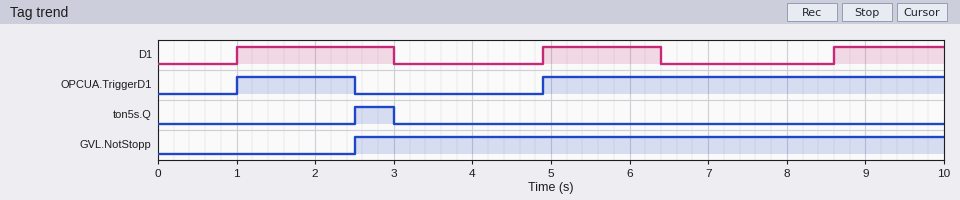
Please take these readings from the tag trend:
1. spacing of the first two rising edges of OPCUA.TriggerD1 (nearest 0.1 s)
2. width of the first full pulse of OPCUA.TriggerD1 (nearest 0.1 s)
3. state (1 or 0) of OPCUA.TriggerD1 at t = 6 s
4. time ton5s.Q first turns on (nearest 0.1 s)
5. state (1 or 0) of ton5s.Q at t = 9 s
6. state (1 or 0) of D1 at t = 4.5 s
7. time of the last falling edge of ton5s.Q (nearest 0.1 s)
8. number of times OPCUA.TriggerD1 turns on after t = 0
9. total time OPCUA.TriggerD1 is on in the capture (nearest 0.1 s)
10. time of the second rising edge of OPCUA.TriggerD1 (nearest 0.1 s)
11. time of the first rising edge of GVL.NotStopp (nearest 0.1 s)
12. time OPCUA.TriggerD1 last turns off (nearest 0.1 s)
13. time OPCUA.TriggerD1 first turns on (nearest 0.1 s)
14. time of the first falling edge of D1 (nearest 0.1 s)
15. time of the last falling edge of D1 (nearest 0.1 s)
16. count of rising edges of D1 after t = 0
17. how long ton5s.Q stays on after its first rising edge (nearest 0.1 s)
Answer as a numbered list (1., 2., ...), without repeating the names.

1. 3.9 s
2. 1.5 s
3. 1
4. 2.5 s
5. 0
6. 0
7. 3.0 s
8. 2
9. 6.6 s
10. 4.9 s
11. 2.5 s
12. 2.5 s
13. 1.0 s
14. 3.0 s
15. 6.4 s
16. 3
17. 0.5 s
